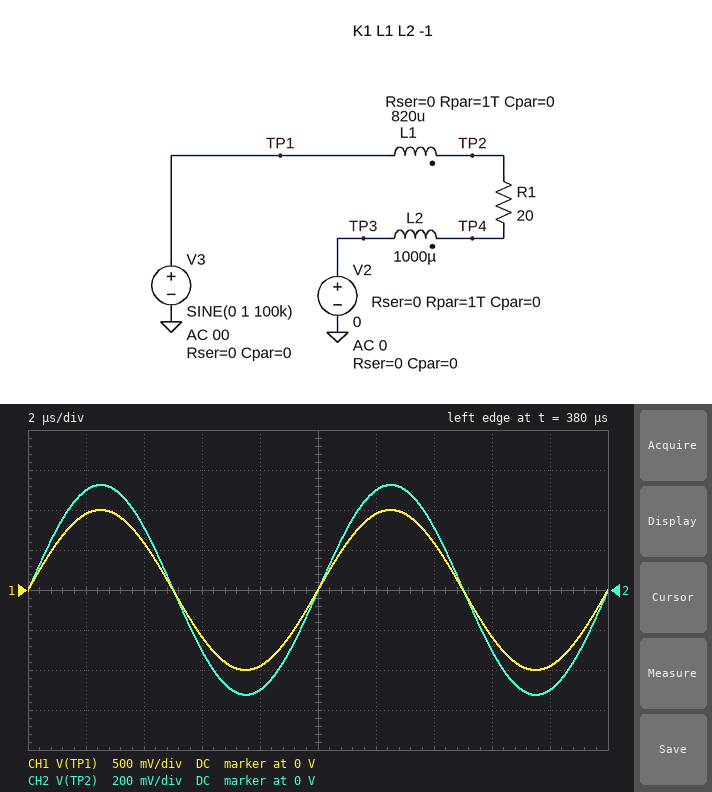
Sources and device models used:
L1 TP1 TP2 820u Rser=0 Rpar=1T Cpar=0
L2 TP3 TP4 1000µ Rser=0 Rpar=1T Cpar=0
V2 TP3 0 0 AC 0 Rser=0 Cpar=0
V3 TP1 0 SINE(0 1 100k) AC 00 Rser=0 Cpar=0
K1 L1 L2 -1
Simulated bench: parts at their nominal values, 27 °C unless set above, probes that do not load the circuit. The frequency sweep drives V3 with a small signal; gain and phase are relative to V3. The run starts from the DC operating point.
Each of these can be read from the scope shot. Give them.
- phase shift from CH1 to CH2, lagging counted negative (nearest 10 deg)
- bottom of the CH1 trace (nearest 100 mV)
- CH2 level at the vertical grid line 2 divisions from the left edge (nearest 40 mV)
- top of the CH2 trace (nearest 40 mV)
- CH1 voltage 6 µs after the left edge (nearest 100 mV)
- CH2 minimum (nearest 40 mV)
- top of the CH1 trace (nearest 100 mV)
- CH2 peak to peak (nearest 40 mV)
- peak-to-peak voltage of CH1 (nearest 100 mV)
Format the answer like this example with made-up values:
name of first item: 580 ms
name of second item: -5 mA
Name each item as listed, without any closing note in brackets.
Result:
phase shift from CH1 to CH2, lagging counted negative: 0 deg
bottom of the CH1 trace: -1.0 V
CH2 level at the vertical grid line 2 divisions from the left edge: 320 mV
top of the CH2 trace: 520 mV
CH1 voltage 6 µs after the left edge: -600 mV
CH2 minimum: -520 mV
top of the CH1 trace: 1.0 V
CH2 peak to peak: 1.04 V
peak-to-peak voltage of CH1: 2.0 V
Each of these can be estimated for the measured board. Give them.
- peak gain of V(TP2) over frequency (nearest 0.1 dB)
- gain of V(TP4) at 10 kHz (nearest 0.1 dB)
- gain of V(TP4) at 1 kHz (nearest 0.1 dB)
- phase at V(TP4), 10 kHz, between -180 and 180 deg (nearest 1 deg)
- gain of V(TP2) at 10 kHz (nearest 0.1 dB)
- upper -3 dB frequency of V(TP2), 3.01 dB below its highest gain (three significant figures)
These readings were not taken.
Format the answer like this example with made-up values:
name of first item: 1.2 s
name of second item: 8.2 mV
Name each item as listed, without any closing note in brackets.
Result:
peak gain of V(TP2) over frequency: 0 dB
gain of V(TP4) at 10 kHz: -5.6 dB
gain of V(TP4) at 1 kHz: -8.1 dB
phase at V(TP4), 10 kHz, between -180 and 180 deg: 5 deg
gain of V(TP2) at 10 kHz: -5.5 dB
upper -3 dB frequency of V(TP2), 3.01 dB below its highest gain: 1.31 kHz
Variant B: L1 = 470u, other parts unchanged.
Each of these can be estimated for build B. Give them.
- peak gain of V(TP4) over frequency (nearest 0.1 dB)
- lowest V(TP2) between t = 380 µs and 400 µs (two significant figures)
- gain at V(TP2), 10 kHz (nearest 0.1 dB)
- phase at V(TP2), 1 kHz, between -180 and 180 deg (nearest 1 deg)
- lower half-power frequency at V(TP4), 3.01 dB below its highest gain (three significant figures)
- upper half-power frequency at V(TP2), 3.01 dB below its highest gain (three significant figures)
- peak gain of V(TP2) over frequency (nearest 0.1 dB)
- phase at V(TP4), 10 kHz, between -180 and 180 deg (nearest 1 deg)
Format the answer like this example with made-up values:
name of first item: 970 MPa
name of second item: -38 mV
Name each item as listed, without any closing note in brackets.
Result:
peak gain of V(TP4) over frequency: -4.5 dB
lowest V(TP2) between t = 380 µs and 400 µs: -590 mV
gain at V(TP2), 10 kHz: -4.4 dB
phase at V(TP2), 1 kHz, between -180 and 180 deg: -14 deg
lower half-power frequency at V(TP4), 3.01 dB below its highest gain: 1.12 kHz
upper half-power frequency at V(TP2), 3.01 dB below its highest gain: 2.06 kHz
peak gain of V(TP2) over frequency: 0 dB
phase at V(TP4), 10 kHz, between -180 and 180 deg: 6 deg
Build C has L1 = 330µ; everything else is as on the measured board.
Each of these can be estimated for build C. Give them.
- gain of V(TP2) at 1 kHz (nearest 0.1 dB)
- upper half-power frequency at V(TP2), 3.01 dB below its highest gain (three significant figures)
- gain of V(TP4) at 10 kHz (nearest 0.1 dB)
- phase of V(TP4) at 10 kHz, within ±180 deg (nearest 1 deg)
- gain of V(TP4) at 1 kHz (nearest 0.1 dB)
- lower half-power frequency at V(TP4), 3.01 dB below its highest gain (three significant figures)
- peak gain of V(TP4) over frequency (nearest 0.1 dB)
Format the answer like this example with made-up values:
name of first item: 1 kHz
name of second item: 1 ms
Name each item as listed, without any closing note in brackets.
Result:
gain of V(TP2) at 1 kHz: -1.1 dB
upper half-power frequency at V(TP2), 3.01 dB below its highest gain: 2.92 kHz
gain of V(TP4) at 10 kHz: -4.0 dB
phase of V(TP4) at 10 kHz, within ±180 deg: 7 deg
gain of V(TP4) at 1 kHz: -8.2 dB
lower half-power frequency at V(TP4), 3.01 dB below its highest gain: 1.28 kHz
peak gain of V(TP4) over frequency: -3.9 dB
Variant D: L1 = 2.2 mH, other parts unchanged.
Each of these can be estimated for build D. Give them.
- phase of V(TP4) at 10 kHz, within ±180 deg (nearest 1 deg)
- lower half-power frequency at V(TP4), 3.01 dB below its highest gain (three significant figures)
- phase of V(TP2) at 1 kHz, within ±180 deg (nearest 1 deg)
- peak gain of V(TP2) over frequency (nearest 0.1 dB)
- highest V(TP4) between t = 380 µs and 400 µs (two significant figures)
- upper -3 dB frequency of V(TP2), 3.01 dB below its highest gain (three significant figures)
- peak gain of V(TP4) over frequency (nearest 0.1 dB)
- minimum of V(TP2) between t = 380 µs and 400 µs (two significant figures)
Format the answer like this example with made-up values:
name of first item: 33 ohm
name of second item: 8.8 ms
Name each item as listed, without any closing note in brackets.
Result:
phase of V(TP4) at 10 kHz, within ±180 deg: 3 deg
lower half-power frequency at V(TP4), 3.01 dB below its highest gain: 516 Hz
phase of V(TP2) at 1 kHz, within ±180 deg: -25 deg
peak gain of V(TP2) over frequency: 0 dB
highest V(TP4) between t = 380 µs and 400 µs: 400 mV
upper -3 dB frequency of V(TP2), 3.01 dB below its highest gain: 628 Hz
peak gain of V(TP4) over frequency: -7.9 dB
minimum of V(TP2) between t = 380 µs and 400 µs: -400 mV
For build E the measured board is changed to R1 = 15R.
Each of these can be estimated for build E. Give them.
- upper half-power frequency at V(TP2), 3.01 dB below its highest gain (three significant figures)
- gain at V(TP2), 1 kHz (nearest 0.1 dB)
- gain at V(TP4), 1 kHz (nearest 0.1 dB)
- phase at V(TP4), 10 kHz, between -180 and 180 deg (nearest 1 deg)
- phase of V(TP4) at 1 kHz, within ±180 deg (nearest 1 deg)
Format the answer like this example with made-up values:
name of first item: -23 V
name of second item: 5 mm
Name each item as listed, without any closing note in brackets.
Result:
upper half-power frequency at V(TP2), 3.01 dB below its highest gain: 981 Hz
gain at V(TP2), 1 kHz: -3.1 dB
gain at V(TP4), 1 kHz: -7.2 dB
phase at V(TP4), 10 kHz, between -180 and 180 deg: 4 deg
phase of V(TP4) at 1 kHz, within ±180 deg: 33 deg
